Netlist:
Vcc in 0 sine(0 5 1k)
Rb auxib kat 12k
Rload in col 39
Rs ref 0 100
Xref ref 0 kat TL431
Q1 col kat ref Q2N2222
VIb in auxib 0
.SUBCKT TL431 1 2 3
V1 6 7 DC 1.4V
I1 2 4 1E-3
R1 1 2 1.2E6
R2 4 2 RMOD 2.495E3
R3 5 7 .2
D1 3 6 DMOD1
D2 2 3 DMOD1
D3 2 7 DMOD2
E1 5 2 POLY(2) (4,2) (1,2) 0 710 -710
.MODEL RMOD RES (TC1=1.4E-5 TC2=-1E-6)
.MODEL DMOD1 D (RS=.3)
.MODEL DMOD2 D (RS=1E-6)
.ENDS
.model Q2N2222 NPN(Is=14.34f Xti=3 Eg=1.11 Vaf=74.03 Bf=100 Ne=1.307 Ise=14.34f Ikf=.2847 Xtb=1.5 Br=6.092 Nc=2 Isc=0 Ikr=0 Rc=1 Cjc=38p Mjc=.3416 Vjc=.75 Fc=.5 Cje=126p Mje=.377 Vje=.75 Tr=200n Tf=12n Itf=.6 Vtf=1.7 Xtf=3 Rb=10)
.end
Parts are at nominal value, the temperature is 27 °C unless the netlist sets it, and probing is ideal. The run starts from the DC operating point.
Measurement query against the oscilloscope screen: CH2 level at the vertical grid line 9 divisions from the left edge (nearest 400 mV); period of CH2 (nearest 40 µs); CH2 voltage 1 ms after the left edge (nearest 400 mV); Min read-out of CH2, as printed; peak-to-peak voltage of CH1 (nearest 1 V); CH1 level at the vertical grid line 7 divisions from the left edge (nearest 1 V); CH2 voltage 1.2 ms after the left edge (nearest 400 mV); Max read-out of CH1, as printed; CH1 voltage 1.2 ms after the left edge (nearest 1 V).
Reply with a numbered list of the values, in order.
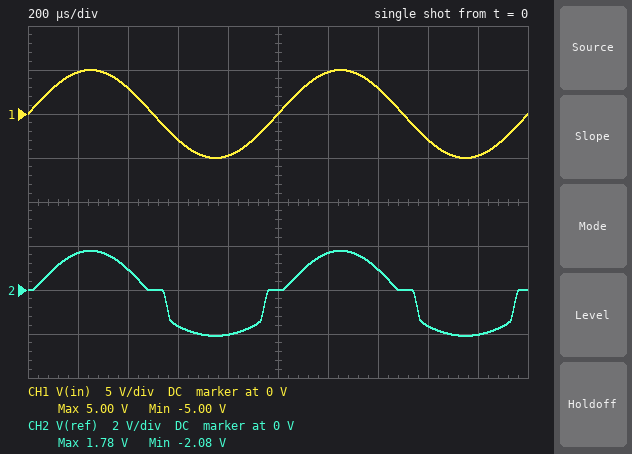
1. -2.0 V
2. 1.00 ms
3. 0 V
4. -2.08 V
5. 10 V
6. 3 V
7. 1.6 V
8. 5.00 V
9. 5 V
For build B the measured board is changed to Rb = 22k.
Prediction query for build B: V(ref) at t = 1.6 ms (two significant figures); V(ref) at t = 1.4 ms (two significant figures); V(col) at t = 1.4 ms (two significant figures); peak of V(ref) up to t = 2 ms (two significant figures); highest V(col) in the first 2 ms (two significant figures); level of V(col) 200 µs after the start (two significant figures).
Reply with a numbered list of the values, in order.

1. -1.6 V
2. 630 mV
3. 2.7 V
4. 1.2 V
5. 4.5 V
6. 4.3 V
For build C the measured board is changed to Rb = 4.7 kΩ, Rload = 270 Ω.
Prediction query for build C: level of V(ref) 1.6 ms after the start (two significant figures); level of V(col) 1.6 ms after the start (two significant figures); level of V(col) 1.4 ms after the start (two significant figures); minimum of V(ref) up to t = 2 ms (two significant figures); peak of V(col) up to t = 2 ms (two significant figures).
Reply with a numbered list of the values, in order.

1. -500 mV
2. -1.4 V
3. 860 mV
4. -1.1 V
5. 1.4 V
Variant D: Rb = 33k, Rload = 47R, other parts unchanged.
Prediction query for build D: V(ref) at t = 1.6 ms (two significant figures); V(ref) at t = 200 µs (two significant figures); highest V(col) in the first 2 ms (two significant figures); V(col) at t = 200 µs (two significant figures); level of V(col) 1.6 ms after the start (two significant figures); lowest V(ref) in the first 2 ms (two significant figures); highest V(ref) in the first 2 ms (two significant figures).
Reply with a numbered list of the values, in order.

1. -1.6 V
2. 850 mV
3. 4.6 V
4. 4.4 V
5. -1.6 V
6. -2.0 V
7. 900 mV
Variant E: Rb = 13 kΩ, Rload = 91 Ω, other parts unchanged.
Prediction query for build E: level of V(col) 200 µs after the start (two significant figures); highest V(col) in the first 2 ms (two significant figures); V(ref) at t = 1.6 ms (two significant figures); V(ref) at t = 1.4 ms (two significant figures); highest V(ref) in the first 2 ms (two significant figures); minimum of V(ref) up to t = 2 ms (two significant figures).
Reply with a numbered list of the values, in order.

1. 3.3 V
2. 3.5 V
3. -1.4 V
4. 890 mV
5. 1.7 V
6. -1.7 V
